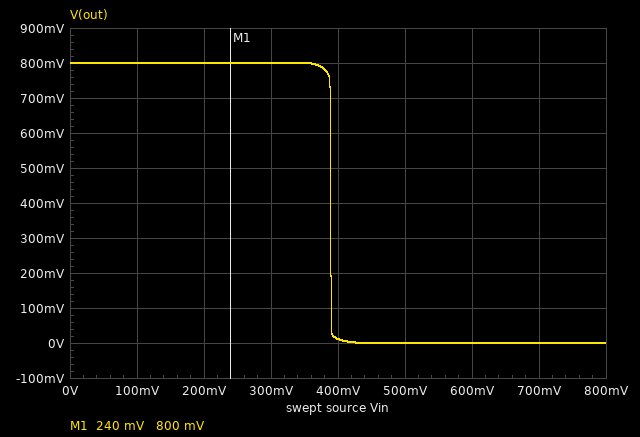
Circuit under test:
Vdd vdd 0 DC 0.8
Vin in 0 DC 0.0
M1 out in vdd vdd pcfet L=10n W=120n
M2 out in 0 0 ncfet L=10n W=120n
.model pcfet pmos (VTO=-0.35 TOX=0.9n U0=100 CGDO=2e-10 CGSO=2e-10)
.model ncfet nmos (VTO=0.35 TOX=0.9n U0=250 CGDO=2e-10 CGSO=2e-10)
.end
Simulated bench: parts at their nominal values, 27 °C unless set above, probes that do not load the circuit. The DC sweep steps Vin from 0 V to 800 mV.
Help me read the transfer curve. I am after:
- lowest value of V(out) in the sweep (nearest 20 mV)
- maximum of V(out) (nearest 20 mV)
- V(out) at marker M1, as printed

0 V
800 mV
800 mV
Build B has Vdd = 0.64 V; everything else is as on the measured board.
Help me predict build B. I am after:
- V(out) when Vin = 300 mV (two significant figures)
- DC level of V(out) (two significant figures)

320 mV
640 mV
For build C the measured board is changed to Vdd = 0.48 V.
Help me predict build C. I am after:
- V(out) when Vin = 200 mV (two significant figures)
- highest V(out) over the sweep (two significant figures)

240 mV
480 mV
